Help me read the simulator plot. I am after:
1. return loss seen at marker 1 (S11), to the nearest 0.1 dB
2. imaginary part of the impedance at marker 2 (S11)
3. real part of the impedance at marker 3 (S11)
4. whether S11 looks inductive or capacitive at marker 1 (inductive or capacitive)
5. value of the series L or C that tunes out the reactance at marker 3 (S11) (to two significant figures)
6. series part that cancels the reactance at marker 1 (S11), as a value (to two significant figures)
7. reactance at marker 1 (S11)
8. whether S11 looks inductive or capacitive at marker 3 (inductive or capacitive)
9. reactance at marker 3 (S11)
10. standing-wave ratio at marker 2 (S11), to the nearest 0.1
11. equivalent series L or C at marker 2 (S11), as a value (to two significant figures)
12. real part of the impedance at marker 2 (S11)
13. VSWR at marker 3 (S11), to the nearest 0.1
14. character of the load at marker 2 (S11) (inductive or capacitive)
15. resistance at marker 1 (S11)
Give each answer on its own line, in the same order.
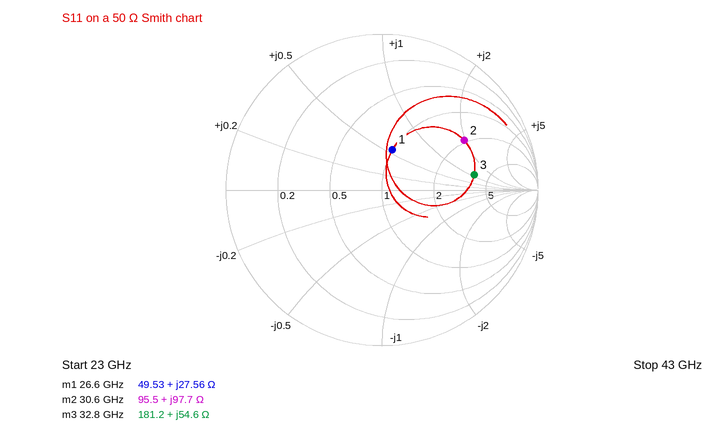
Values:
11.5 dB
+97.7 Ω
181.2 Ω
inductive
89 fF
220 fF
+27.56 Ω
inductive
+54.6 Ω
4.2
510 pH
95.5 Ω
4.0
inductive
49.53 Ω
